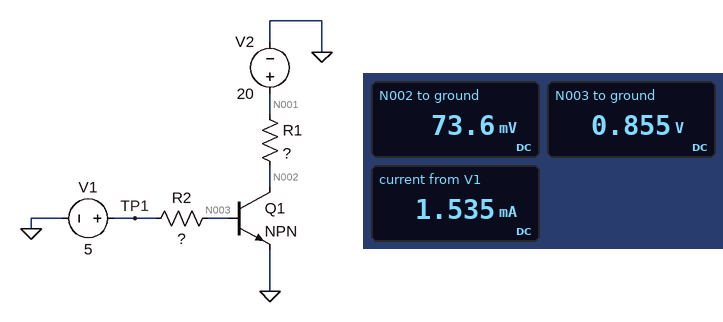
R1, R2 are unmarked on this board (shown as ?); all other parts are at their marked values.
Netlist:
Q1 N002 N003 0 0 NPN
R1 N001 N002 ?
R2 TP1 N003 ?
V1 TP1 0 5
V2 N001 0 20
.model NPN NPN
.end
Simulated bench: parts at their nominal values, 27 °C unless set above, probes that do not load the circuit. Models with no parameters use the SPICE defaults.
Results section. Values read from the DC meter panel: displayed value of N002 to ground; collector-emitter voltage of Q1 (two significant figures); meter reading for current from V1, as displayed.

73.6 mV
74 mV
1.535 mA
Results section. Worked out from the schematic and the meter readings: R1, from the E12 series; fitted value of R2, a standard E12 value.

1 kΩ
2.7 kΩ
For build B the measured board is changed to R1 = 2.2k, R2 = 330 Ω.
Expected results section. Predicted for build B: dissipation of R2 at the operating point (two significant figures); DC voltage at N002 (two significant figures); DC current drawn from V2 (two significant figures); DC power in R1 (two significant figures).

52 mW
26 mV
9.1 mA
180 mW
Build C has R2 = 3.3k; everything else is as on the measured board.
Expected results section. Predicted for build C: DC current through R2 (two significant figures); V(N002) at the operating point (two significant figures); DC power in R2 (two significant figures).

1.3 mA
79 mV
5.2 mW
